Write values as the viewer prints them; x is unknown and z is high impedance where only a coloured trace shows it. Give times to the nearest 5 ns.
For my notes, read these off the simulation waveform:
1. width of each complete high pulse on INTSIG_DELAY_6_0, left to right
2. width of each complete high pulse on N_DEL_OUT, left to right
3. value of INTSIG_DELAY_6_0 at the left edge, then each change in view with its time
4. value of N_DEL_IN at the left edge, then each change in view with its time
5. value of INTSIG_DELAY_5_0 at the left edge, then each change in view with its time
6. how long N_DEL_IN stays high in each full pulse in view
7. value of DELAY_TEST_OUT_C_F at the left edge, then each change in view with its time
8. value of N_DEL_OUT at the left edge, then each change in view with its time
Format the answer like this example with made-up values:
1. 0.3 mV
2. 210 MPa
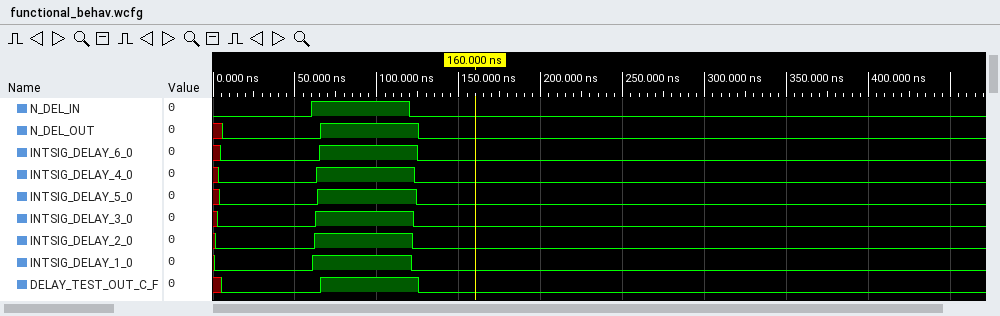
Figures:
1. 60 ns
2. 60 ns
3. x, 0 at 5 ns, 1 at 65 ns, 0 at 125 ns
4. 0, 1 at 60 ns, 0 at 120 ns
5. x, 0 at 5 ns, 1 at 65 ns, 0 at 125 ns
6. 60 ns
7. x, 0 at 5 ns, 1 at 65 ns, 0 at 125 ns
8. x, 0 at 5 ns, 1 at 65 ns, 0 at 125 ns
